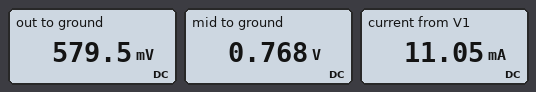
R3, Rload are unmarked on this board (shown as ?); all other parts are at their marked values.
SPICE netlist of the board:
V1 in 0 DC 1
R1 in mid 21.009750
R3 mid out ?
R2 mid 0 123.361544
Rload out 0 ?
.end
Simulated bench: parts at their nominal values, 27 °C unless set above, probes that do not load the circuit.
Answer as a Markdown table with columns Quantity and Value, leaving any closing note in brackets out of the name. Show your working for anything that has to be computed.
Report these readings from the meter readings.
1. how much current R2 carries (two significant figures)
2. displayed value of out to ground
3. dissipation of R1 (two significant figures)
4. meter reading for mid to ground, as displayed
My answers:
| Quantity | Value |
|---|---|
| how much current R2 carries | (768 mV) / 123.4 Ω = 6.2 mA |
| displayed value of out to ground | 579.5 mV |
| dissipation of R1 | (1 V - 768 mV)^2 / 21.01 Ω = 2.6 mW |
| meter reading for mid to ground, as displayed | 0.768 V |
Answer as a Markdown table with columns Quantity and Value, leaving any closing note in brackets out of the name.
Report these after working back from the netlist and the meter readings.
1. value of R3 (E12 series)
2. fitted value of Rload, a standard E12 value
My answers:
| Quantity | Value |
|---|---|
| value of R3 | 39 Ω |
| fitted value of Rload, a standard E12 value | 120 Ω |
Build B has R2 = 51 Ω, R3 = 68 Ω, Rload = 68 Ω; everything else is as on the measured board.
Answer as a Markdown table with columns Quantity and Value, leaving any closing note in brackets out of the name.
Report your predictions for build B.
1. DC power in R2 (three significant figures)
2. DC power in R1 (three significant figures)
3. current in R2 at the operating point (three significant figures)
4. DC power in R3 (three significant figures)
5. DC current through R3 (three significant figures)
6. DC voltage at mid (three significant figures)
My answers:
| Quantity | Value |
|---|---|
| DC power in R2 | 7.99 mW |
| DC power in R1 | 6.22 mW |
| current in R2 at the operating point | 12.5 mA |
| DC power in R3 | 1.50 mW |
| DC current through R3 | 4.69 mA |
| DC voltage at mid | 638 mV |
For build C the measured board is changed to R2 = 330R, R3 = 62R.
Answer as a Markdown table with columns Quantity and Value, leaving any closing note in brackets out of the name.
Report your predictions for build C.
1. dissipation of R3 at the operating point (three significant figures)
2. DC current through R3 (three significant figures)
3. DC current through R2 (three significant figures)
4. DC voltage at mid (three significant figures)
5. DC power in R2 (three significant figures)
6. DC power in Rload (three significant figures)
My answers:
| Quantity | Value |
|---|---|
| dissipation of R3 at the operating point | 1.35 mW |
| DC current through R3 | 4.66 mA |
| DC current through R2 | 2.57 mA |
| DC voltage at mid | 848 mV |
| DC power in R2 | 2.18 mW |
| DC power in Rload | 2.61 mW |
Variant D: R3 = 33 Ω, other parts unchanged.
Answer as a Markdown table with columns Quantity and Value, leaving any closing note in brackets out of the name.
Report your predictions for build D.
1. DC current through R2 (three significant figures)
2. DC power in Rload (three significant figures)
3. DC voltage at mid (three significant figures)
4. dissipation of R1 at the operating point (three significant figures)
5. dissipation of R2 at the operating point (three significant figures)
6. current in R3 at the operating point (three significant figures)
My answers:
| Quantity | Value |
|---|---|
| DC current through R2 | 6.20 mA |
| DC power in Rload | 3.00 mW |
| DC voltage at mid | 765 mV |
| dissipation of R1 at the operating point | 2.63 mW |
| dissipation of R2 at the operating point | 4.74 mW |
| current in R3 at the operating point | 5.00 mA |
